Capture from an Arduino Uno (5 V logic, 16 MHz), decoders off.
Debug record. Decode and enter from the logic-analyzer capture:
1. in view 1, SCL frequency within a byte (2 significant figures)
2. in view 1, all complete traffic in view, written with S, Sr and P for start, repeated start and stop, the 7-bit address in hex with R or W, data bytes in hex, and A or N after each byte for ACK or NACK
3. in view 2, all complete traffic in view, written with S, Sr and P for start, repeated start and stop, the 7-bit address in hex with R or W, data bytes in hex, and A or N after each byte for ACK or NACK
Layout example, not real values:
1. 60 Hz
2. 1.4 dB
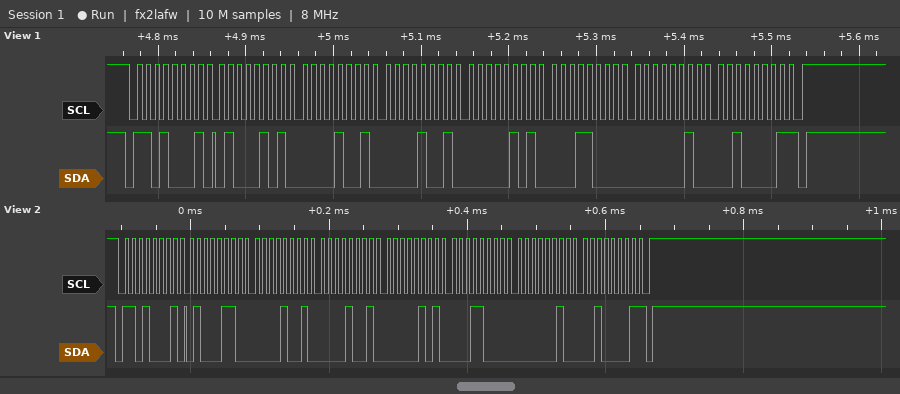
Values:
1. 100 kHz
2. S 68R A 45 A 09 A 09 A 05 A 18 A 02 A 21 N P
3. S 68R A 46 A 09 A 09 A 05 A 18 A 02 A 21 N P
